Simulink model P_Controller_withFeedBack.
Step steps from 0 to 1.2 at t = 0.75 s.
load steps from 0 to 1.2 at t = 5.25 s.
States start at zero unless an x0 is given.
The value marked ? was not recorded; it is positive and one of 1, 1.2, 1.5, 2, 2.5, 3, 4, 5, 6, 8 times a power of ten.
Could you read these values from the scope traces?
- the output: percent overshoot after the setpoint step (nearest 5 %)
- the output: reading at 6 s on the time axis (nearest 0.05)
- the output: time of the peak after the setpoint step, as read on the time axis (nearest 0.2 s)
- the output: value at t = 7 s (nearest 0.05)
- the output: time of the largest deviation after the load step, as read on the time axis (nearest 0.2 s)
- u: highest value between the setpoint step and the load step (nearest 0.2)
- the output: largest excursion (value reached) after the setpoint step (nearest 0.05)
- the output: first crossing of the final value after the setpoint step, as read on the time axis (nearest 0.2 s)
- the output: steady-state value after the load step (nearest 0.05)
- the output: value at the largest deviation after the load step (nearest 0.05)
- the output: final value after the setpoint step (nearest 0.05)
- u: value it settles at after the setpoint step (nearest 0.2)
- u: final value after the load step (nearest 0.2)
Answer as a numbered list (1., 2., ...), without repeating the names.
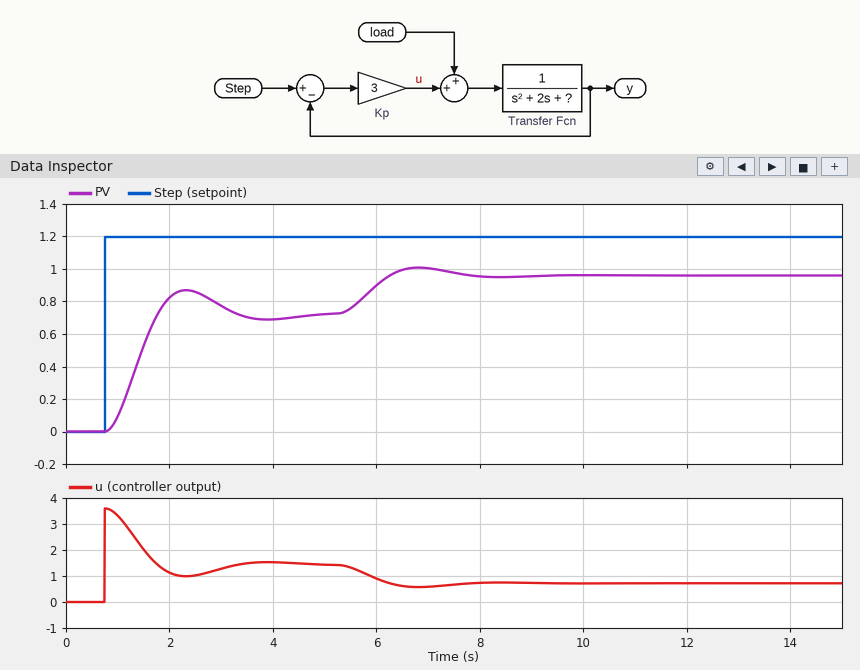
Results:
1. 20 %
2. 0.90
3. 2.4 s
4. 1.00
5. 6.8 s
6. 3.6
7. 0.85
8. 1.8 s
9. 0.95
10. 1.00
11. 0.70
12. 1.4
13. 0.8
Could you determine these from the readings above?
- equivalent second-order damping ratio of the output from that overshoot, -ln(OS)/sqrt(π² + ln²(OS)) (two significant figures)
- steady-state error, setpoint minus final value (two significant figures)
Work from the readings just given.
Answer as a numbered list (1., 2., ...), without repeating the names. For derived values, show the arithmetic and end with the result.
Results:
1. ln(0.2) = -1.609; 1.609 / sqrt(9.870 + 2.590) = 0.46
2. 1.2 - 0.7 = 0.50
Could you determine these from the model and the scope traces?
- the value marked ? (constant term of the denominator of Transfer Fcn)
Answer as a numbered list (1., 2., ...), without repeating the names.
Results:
1. 2
